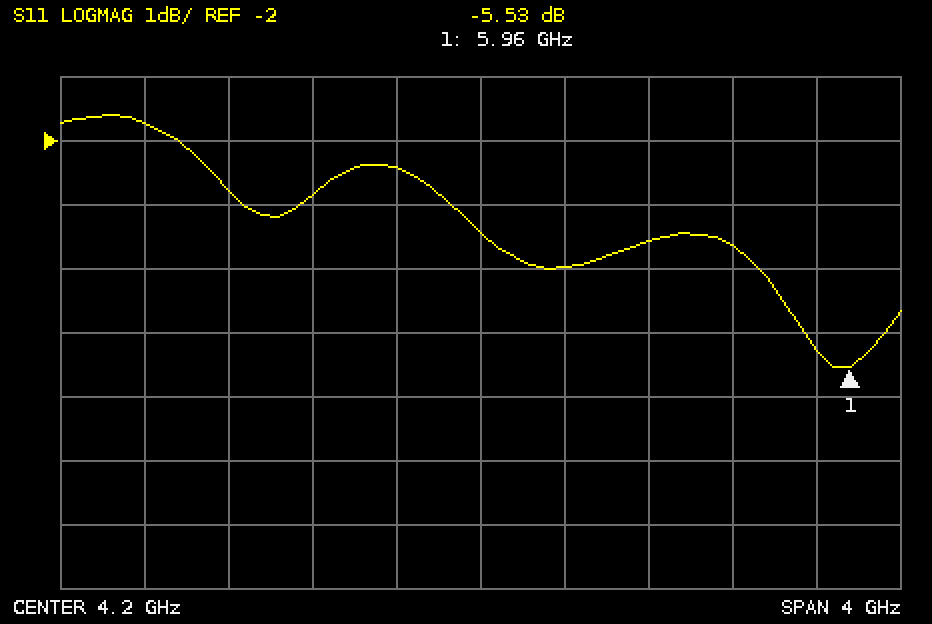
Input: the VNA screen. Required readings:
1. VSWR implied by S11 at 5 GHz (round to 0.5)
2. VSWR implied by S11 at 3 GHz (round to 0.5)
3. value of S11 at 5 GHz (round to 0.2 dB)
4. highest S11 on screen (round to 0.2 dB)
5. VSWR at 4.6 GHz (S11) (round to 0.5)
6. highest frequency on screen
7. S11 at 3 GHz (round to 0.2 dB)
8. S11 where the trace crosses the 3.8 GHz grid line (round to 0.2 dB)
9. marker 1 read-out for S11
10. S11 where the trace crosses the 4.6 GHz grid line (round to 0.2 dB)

5.0
6.5
-3.6 dB
-1.6 dB
4.5
6.2 GHz
-2.8 dB
-2.4 dB
-5.53 dB
-4.0 dB
